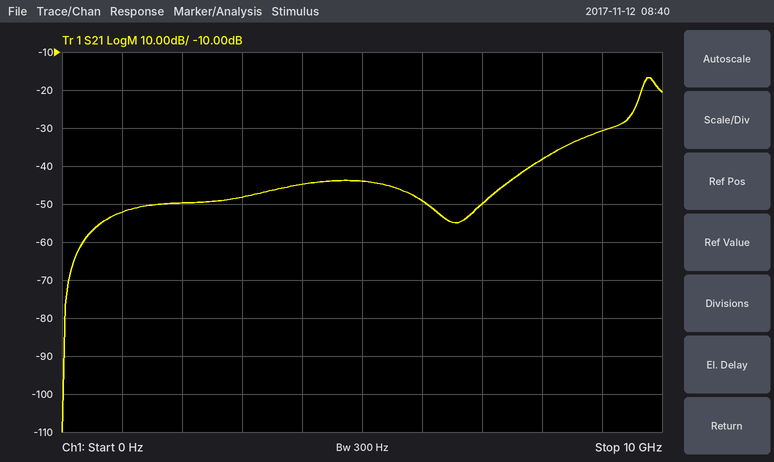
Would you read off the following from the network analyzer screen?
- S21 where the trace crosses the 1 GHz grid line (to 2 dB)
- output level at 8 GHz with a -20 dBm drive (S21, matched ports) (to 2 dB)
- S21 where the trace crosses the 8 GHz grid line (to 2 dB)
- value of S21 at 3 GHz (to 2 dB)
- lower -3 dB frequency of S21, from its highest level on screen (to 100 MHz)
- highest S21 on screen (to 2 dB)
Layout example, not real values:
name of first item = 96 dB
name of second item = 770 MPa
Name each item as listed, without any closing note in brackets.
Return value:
S21 where the trace crosses the 1 GHz grid line = -52 dB
output level at 8 GHz with a -20 dBm drive (S21, matched ports) = -58 dBm
S21 where the trace crosses the 8 GHz grid line = -38 dB
value of S21 at 3 GHz = -48 dB
lower -3 dB frequency of S21, from its highest level on screen = 9.7 GHz
highest S21 on screen = -16 dB
